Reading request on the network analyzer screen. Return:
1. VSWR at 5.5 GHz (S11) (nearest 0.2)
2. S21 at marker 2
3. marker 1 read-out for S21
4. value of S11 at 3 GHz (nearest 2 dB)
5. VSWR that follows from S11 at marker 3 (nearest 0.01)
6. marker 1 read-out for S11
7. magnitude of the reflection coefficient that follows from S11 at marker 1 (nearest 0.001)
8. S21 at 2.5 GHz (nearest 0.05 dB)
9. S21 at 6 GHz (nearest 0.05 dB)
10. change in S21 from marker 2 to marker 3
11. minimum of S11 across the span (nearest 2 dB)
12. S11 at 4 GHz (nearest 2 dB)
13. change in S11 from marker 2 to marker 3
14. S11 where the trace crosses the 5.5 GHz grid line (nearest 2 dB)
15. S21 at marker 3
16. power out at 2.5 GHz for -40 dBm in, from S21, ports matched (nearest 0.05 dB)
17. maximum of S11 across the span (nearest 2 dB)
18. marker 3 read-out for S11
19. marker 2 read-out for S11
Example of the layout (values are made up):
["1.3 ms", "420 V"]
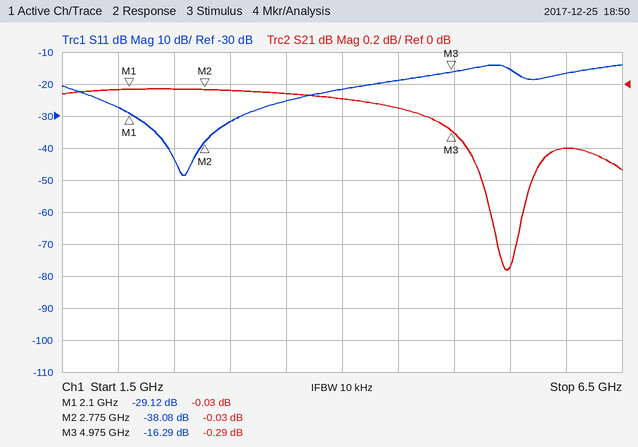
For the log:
["1.4", "-0.03 dB", "-0.03 dB", "-32 dB", "1.36", "-29.12 dB", "0.035", "-0.05 dB", "-0.40 dB", "-0.26 dB", "-48 dB", "-22 dB", "21.79 dB", "-16 dB", "-0.29 dB", "-40.05 dBm", "-14 dB", "-16.29 dB", "-38.08 dB"]
